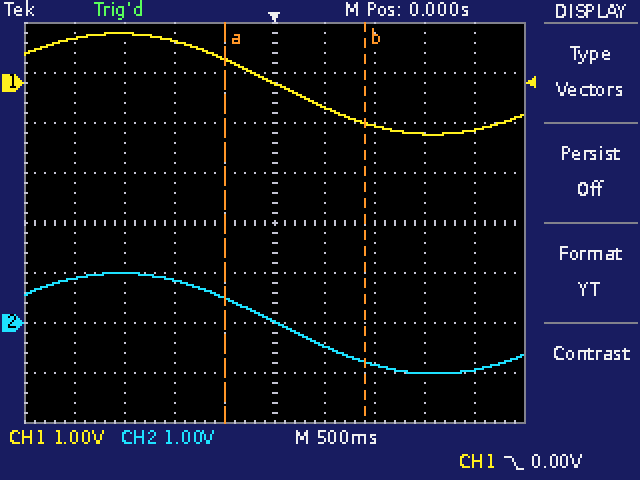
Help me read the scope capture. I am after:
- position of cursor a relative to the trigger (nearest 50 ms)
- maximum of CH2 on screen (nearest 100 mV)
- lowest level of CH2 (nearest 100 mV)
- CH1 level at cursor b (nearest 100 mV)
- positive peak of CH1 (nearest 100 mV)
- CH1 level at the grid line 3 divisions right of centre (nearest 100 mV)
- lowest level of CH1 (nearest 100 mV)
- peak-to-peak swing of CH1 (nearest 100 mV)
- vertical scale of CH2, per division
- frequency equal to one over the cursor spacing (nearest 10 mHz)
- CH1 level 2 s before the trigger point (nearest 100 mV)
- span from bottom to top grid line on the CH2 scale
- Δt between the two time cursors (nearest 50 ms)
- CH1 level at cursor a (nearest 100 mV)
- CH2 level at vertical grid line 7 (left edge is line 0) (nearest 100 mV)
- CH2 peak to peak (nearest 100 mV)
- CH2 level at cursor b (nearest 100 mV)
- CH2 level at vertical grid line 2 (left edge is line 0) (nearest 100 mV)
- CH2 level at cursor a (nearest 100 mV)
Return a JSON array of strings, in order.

["-500 ms", "1.0 V", "-1.0 V", "-800 mV", "1.0 V", "-1.0 V", "-1.0 V", "2.0 V", "1 V", "710 mHz", "900 mV", "8 V", "1.40 s", "500 mV", "-800 mV", "2.0 V", "-800 mV", "1.0 V", "500 mV"]
